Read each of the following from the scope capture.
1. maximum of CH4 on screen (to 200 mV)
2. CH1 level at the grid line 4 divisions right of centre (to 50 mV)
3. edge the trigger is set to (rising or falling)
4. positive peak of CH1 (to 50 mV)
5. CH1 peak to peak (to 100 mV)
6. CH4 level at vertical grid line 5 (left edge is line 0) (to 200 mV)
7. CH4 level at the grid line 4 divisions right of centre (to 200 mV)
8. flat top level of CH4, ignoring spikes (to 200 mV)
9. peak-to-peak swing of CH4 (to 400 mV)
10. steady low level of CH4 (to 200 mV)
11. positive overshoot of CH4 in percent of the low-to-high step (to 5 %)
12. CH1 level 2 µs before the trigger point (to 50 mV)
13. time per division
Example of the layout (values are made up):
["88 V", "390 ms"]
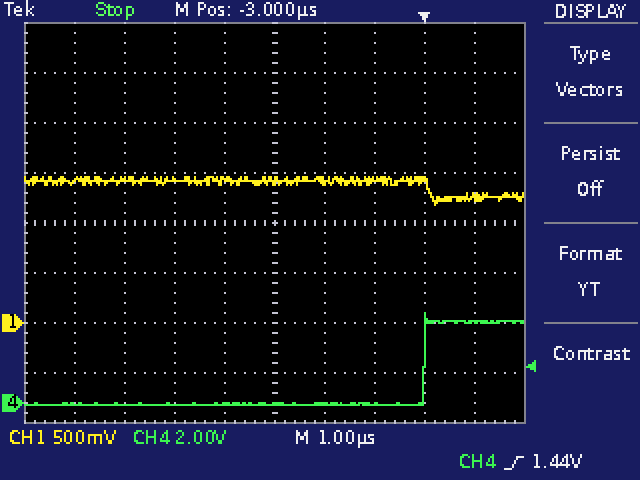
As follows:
["3.6 V", "1.25 V", "rising", "1.45 V", "300 mV", "0.0 V", "3.2 V", "3.2 V", "3.6 V", "0.0 V", "10 %", "1.40 V", "1 µs"]
